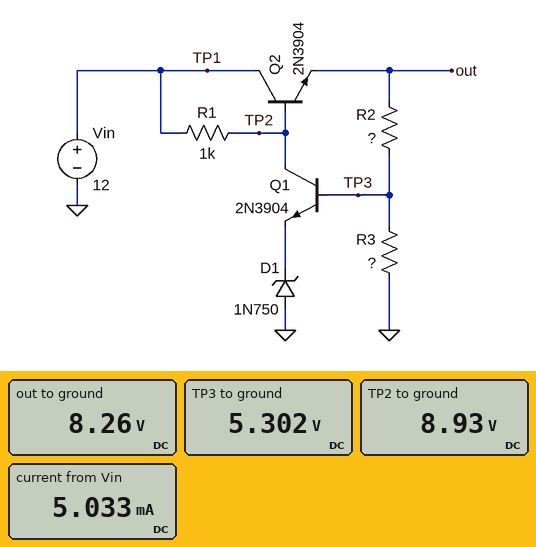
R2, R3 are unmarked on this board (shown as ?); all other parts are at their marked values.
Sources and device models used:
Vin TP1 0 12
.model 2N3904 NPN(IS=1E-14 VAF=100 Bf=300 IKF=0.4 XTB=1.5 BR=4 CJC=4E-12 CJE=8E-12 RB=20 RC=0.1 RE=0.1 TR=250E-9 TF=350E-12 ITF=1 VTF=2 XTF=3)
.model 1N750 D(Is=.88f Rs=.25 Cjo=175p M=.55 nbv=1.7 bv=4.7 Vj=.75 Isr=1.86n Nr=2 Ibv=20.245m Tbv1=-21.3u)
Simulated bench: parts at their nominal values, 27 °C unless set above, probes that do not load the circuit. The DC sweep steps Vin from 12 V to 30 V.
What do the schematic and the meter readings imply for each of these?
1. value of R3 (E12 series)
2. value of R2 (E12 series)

2.7 kΩ
1.5 kΩ
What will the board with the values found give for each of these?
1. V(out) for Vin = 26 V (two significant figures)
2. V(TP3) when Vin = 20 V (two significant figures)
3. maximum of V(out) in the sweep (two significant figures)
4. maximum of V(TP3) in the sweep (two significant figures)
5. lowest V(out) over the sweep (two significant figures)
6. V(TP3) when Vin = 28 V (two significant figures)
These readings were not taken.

8.5 V
5.4 V
8.6 V
5.4 V
8.3 V
5.4 V
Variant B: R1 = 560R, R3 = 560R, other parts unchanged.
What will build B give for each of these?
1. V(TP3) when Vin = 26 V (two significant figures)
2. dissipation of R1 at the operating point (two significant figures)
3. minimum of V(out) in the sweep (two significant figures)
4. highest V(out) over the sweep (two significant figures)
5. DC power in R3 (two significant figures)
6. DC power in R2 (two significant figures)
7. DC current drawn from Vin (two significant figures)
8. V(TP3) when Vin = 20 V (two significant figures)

5.4 V
190 nW
11 V
20 V
17 mW
45 mW
5.5 mA
5.2 V
